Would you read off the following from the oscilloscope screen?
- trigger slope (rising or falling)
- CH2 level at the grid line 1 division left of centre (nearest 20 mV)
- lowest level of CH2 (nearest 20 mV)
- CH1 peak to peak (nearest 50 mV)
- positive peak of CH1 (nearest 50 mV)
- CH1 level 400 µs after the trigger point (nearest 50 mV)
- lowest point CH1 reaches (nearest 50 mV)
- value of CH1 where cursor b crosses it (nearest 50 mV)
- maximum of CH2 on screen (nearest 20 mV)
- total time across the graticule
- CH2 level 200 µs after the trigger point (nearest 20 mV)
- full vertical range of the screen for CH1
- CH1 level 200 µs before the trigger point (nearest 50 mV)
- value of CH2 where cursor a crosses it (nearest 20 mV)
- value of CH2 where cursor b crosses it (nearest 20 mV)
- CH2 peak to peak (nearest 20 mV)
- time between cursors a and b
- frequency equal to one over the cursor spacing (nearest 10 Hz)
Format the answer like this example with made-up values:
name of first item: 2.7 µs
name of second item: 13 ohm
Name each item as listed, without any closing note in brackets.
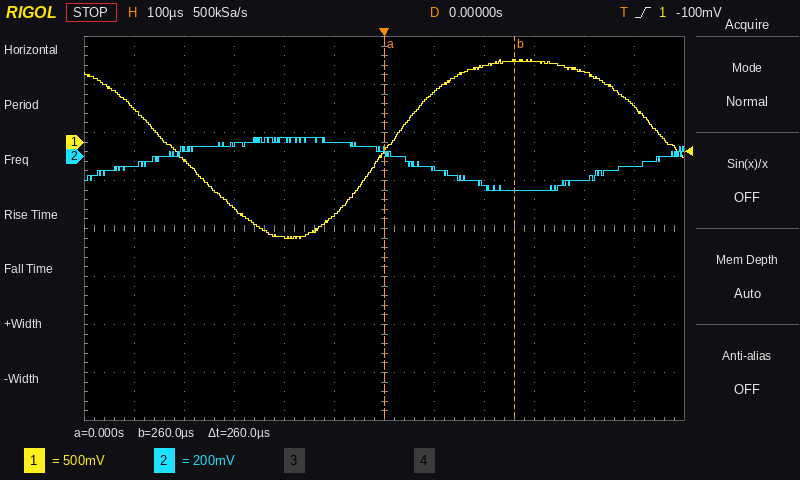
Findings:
trigger slope: rising
CH2 level at the grid line 1 division left of centre: 60 mV
lowest level of CH2: -140 mV
CH1 peak to peak: 1.85 V
positive peak of CH1: 850 mV
CH1 level 400 µs after the trigger point: 750 mV
lowest point CH1 reaches: -1.00 V
value of CH1 where cursor b crosses it: 850 mV
maximum of CH2 on screen: 80 mV
total time across the graticule: 1.2 ms
CH2 level 200 µs after the trigger point: -120 mV
full vertical range of the screen for CH1: 4 V
CH1 level 200 µs before the trigger point: -1.00 V
value of CH2 where cursor a crosses it: 20 mV
value of CH2 where cursor b crosses it: -140 mV
CH2 peak to peak: 220 mV
time between cursors a and b: 260 µs
frequency equal to one over the cursor spacing: 3.85 kHz
